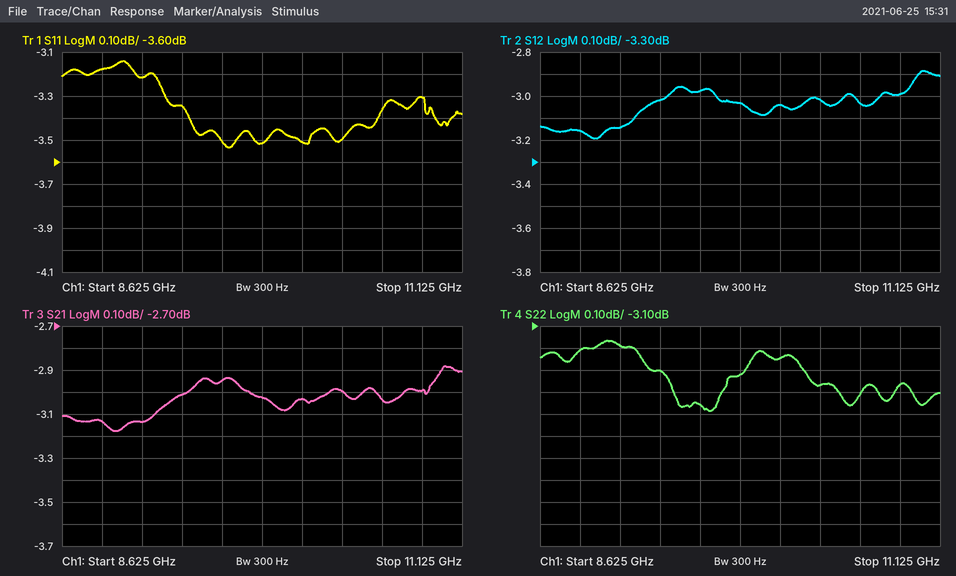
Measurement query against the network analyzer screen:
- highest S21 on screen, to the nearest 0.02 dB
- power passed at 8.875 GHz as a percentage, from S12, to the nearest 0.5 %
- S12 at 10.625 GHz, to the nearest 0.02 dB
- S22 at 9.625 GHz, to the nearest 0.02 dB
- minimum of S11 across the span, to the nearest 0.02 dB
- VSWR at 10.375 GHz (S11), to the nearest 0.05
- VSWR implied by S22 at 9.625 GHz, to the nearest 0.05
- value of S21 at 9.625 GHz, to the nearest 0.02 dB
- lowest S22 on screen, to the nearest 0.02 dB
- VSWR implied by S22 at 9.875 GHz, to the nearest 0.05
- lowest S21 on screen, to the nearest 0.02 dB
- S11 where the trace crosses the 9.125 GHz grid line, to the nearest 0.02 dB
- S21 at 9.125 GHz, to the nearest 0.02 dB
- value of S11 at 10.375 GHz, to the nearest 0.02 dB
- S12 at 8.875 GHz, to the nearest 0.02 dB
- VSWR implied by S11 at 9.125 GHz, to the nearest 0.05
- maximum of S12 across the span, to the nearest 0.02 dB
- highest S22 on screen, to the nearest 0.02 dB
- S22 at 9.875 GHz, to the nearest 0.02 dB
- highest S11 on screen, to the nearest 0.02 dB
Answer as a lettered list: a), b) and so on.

a) -2.88 dB
b) 48.5 %
c) -3.04 dB
d) -3.46 dB
e) -3.54 dB
f) 5.05
g) 5.10
h) -2.94 dB
i) -3.48 dB
j) 5.30
k) -3.18 dB
l) -3.22 dB
m) -3.14 dB
n) -3.50 dB
o) -3.16 dB
p) 5.45
q) -2.88 dB
r) -3.16 dB
s) -3.32 dB
t) -3.14 dB
